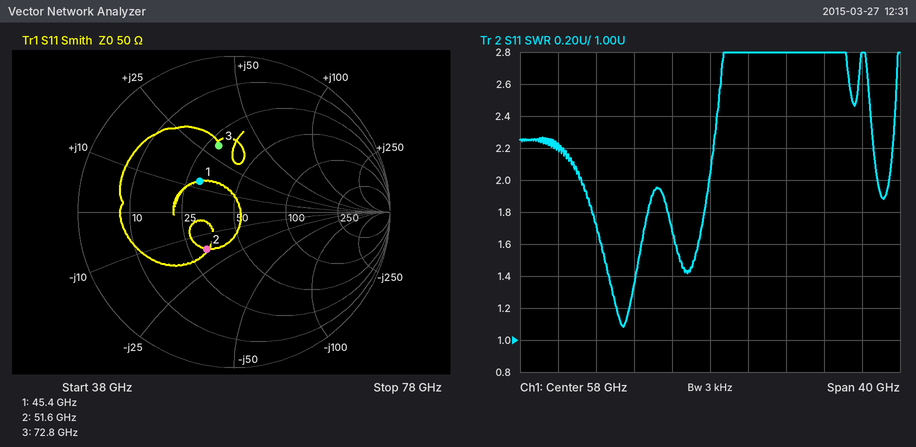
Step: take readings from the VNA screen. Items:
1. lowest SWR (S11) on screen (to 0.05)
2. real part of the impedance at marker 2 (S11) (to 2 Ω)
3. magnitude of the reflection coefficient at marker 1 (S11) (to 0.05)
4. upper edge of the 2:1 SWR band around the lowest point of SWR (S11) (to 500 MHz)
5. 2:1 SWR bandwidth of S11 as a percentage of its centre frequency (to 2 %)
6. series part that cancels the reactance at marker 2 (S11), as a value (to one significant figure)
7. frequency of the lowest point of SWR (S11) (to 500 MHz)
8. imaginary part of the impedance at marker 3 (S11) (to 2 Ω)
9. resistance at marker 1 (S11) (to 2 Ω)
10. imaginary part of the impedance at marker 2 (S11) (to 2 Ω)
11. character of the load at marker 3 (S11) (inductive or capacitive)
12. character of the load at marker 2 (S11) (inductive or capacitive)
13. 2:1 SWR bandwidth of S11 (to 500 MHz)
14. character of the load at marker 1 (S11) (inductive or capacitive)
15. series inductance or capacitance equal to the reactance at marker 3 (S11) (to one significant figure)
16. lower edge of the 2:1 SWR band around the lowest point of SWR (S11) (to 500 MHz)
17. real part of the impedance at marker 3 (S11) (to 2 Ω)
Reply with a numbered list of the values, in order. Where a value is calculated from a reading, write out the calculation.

1. 1.10
2. 32 Ω
3. 0.30
4. 58.0 GHz
5. 13.5 GHz / 51.25 GHz ≈ 26 %
6. L = 16 Ω/(2π × 51.6 GHz) ≈ 49.4 pH, so 50 pH to one significant figure
7. 49.0 GHz
8. +30 Ω
9. 30 Ω
10. -16 Ω
11. inductive
12. capacitive
13. 58.0 GHz − 44.5 GHz = 13.5 GHz
14. inductive
15. L = 30 Ω/(2π × 72.8 GHz) ≈ 65.6 pH, so 70 pH to one significant figure
16. 44.5 GHz
17. 30 Ω
